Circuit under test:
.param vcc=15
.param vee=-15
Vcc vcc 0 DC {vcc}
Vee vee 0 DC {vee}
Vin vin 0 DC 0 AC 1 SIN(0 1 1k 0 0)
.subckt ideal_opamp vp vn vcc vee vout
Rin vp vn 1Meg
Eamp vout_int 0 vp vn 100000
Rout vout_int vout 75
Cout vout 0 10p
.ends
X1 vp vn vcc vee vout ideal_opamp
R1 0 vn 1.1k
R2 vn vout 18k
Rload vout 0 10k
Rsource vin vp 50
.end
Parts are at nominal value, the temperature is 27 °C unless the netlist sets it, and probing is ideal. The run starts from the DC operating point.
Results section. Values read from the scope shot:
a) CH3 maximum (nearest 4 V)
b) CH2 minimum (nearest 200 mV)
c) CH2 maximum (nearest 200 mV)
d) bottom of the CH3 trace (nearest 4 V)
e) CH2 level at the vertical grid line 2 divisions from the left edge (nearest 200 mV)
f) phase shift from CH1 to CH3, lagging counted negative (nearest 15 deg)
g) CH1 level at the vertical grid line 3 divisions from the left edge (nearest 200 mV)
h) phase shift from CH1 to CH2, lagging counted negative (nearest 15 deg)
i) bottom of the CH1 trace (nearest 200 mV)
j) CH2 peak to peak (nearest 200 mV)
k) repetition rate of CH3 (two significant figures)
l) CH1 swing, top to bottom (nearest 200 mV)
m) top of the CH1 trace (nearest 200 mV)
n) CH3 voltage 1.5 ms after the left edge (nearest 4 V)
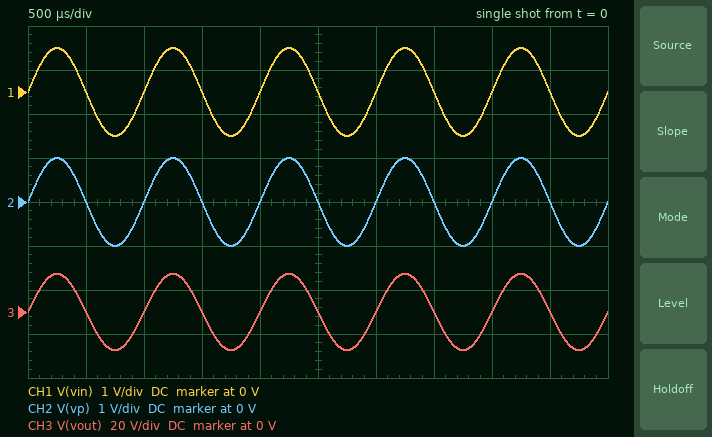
16 V
-1.0 V
1.0 V
-16 V
0 V
0 deg
0 V
0 deg
-1.0 V
2.0 V
1.0 kHz
2.0 V
1.0 V
0 V
